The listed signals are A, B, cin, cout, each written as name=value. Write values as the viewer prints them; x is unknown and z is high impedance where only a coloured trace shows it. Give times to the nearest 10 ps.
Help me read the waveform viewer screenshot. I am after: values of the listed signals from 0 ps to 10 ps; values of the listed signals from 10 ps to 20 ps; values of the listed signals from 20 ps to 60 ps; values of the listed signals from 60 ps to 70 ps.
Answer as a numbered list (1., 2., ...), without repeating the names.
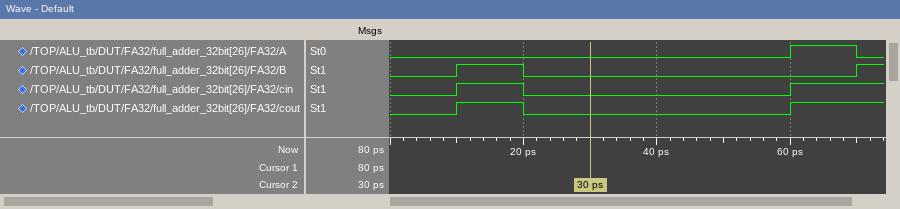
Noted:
1. A=0, B=0, cin=0, cout=0
2. A=0, B=1, cin=1, cout=1
3. A=0, B=0, cin=0, cout=0
4. A=1, B=0, cin=1, cout=1
